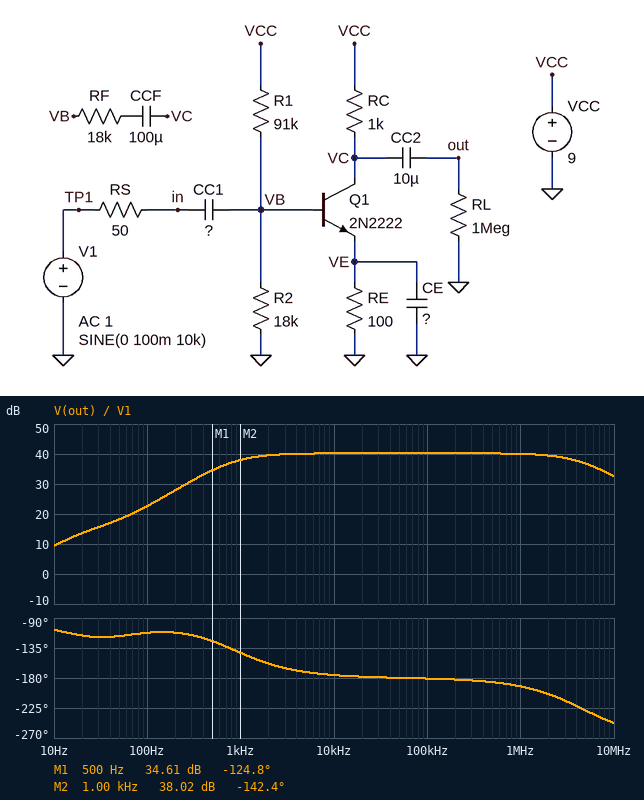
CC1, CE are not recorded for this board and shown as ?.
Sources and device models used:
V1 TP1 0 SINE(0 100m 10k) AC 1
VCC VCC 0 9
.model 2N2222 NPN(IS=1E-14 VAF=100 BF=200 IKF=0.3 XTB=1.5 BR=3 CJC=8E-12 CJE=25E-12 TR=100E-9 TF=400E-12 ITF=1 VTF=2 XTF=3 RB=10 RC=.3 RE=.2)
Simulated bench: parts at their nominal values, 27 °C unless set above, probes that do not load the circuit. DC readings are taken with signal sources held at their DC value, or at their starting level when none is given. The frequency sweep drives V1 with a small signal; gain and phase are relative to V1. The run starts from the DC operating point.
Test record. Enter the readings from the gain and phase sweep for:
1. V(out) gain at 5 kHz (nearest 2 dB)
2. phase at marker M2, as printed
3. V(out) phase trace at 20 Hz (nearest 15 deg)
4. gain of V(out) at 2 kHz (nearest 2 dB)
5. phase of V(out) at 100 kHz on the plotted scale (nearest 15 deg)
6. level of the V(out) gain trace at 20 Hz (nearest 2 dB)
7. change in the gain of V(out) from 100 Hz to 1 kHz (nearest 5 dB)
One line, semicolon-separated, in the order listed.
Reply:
40 dB; -142.4 deg; -120 deg; 40 dB; -180 deg; 14 dB; 15 dB
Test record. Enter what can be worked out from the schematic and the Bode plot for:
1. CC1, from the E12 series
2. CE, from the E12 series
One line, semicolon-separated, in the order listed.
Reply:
3.9 µF; 33 µF
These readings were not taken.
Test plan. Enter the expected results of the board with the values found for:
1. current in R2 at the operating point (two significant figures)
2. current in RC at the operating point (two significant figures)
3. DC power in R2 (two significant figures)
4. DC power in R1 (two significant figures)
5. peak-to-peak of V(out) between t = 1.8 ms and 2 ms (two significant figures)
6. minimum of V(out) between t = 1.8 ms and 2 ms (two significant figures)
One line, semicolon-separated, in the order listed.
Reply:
64 µA; 4.5 mA; 74 µW; 680 µW; 8.2 V; -4.0 V
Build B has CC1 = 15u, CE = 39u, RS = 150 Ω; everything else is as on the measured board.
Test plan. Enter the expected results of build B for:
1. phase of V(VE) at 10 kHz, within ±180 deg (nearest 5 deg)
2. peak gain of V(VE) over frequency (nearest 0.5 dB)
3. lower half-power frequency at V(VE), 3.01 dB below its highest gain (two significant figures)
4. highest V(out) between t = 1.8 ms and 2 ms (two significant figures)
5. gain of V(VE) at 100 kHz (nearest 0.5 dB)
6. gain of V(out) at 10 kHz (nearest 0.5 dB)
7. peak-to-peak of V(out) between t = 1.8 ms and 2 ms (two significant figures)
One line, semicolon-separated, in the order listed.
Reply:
-90 deg; -2.5 dB; 5.6 Hz; 4.0 V; -51.5 dB; 36.0 dB; 7.9 V
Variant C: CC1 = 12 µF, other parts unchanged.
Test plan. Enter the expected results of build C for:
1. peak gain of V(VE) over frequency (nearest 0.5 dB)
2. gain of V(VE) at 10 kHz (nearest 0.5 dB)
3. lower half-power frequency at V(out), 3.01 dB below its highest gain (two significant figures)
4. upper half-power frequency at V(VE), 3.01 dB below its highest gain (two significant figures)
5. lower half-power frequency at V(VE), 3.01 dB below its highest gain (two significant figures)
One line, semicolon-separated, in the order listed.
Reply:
-2.0 dB; -25.5 dB; 650 Hz; 670 Hz; 7.4 Hz
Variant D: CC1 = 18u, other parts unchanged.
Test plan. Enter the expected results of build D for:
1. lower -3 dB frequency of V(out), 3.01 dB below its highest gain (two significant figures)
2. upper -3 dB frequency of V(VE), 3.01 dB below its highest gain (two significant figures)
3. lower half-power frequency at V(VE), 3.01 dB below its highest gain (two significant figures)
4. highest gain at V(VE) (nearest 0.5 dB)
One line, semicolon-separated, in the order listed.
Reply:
630 Hz; 640 Hz; 5.2 Hz; -1.5 dB
